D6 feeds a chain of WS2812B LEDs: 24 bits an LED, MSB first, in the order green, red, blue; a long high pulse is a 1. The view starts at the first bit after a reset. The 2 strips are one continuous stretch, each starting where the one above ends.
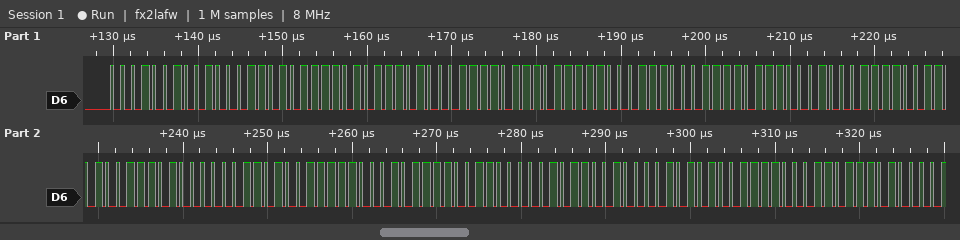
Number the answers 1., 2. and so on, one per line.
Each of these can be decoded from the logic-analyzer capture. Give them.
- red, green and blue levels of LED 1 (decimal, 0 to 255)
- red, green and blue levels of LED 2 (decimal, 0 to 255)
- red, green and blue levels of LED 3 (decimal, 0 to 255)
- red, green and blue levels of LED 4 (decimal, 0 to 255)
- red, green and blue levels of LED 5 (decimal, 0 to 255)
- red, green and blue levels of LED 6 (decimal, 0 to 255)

1. 70, 18, 189
2. 123, 116, 190
3. 247, 56, 17
4. 157, 230, 3
5. 139, 79, 204
6. 66, 22, 167
